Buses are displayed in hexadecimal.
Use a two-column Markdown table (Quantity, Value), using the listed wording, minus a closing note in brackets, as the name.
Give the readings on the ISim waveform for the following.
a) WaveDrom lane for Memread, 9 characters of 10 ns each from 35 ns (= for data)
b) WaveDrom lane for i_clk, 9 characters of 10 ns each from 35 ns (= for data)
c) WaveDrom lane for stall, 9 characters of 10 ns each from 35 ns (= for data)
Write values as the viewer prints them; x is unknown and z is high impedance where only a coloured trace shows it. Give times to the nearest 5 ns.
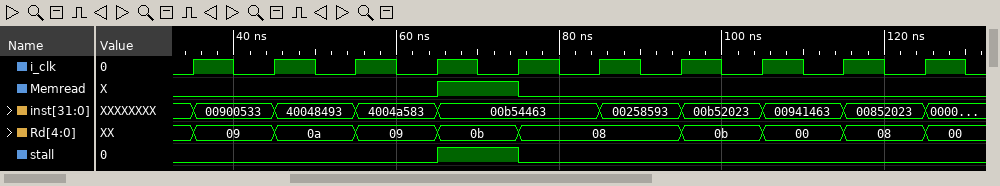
| Quantity | Value |
|---|---|
| WaveDrom lane for Memread, 9 characters of 10 ns each from 35 ns | {name: 'Memread', wave: '0..10....'} |
| WaveDrom lane for i_clk, 9 characters of 10 ns each from 35 ns | {name: 'i_clk', wave: 'p........'} |
| WaveDrom lane for stall, 9 characters of 10 ns each from 35 ns | {name: 'stall', wave: '0..10....'} |
